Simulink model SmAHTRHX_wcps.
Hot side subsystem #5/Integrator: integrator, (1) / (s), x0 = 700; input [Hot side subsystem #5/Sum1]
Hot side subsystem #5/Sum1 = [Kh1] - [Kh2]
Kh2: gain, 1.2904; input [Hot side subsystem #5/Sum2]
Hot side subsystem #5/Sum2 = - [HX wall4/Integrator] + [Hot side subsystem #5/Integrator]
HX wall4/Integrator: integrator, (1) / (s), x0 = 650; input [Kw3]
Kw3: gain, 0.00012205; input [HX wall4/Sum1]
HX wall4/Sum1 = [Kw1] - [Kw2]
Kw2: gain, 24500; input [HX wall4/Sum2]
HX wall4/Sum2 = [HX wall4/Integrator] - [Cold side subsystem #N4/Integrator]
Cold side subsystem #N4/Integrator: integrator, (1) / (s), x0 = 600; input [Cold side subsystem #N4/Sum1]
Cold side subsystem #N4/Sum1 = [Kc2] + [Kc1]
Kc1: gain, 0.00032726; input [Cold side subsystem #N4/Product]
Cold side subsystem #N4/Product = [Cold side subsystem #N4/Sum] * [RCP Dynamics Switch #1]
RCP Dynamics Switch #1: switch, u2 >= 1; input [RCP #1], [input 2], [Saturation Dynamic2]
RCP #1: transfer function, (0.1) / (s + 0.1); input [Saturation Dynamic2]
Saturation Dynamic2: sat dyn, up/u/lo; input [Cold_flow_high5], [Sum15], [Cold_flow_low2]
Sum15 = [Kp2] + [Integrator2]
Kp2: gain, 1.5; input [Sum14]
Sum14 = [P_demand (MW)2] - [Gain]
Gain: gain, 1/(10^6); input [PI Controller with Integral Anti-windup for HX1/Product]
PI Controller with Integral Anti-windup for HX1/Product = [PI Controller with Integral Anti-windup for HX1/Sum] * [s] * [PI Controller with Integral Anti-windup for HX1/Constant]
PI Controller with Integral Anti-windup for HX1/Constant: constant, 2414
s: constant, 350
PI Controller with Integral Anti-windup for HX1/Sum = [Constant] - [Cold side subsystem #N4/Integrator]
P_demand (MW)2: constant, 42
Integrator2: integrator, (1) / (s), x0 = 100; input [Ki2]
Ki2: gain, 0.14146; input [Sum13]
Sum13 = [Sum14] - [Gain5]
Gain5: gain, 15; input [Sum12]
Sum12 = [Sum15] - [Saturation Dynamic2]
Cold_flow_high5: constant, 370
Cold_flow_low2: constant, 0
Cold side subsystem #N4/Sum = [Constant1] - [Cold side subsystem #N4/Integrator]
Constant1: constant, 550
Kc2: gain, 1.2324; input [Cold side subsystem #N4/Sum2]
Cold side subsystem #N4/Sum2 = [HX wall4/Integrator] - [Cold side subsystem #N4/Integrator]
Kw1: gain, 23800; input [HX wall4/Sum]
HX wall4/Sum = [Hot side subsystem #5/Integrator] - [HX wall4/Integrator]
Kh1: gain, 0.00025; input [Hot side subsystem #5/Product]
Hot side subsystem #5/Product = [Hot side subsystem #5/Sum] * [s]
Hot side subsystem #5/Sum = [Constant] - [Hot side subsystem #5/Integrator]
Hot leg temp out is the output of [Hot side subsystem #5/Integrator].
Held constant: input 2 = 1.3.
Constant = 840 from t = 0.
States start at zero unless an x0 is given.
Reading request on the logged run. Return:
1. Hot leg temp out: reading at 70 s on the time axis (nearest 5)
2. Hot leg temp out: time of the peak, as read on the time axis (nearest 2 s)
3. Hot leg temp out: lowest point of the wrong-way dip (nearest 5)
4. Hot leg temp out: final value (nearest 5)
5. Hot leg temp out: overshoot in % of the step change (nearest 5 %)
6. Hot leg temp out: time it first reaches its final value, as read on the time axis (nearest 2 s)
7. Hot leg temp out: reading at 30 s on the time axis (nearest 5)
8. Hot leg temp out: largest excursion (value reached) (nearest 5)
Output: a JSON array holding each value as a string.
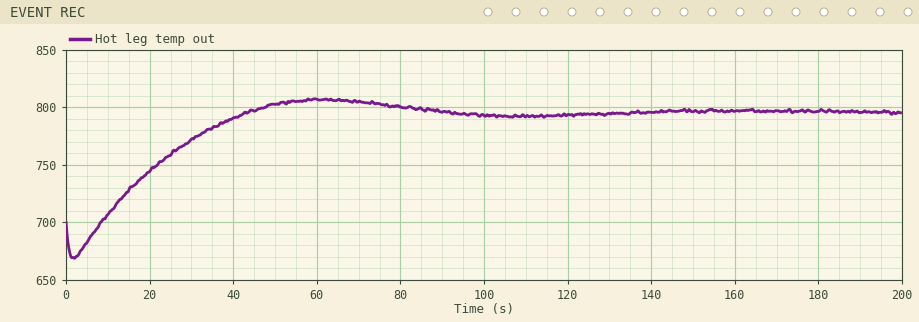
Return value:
["805", "62 s", "670", "795", "10 %", "44 s", "770", "805"]
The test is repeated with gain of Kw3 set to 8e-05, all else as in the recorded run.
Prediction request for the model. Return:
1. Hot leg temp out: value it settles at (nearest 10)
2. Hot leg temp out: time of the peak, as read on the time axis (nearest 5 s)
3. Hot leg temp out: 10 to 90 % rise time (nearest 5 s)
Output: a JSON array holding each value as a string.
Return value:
["800", "65 s", "30 s"]
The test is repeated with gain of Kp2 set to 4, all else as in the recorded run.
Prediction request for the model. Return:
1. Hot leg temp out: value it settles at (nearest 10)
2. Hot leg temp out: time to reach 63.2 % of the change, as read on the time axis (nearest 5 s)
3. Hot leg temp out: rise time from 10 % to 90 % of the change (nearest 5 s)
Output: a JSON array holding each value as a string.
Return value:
["800", "35 s", "65 s"]
